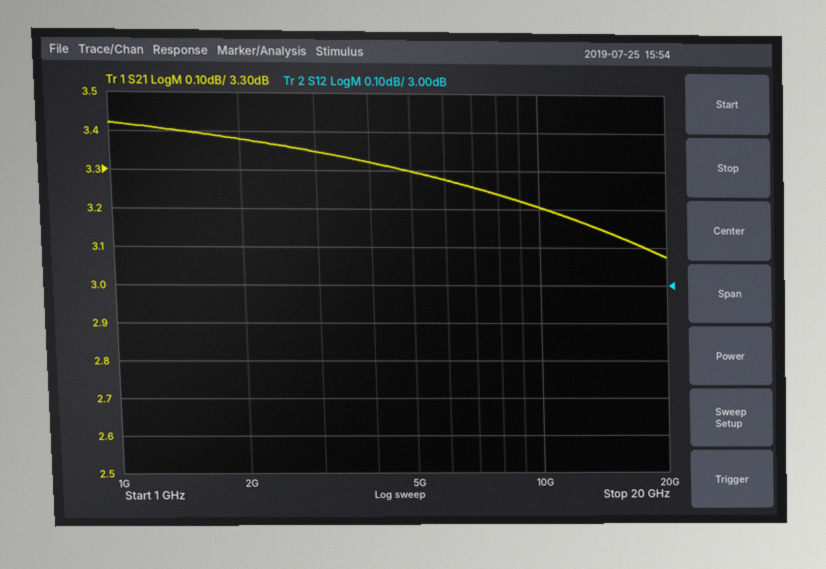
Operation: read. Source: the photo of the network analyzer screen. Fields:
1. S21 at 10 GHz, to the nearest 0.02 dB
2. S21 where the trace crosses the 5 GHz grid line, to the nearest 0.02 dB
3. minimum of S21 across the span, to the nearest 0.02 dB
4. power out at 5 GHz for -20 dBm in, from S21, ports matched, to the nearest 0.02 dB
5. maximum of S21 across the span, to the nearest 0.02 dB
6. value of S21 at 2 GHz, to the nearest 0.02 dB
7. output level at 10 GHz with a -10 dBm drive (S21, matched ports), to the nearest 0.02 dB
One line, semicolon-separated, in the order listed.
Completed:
3.20 dB; 3.30 dB; 3.08 dB; -16.70 dBm; 3.42 dB; 3.38 dB; -6.80 dBm
